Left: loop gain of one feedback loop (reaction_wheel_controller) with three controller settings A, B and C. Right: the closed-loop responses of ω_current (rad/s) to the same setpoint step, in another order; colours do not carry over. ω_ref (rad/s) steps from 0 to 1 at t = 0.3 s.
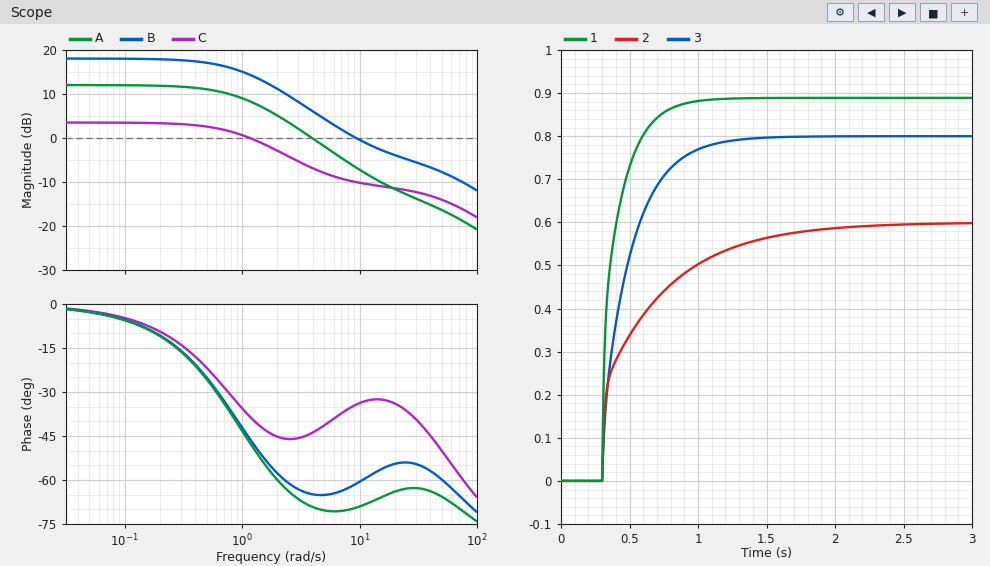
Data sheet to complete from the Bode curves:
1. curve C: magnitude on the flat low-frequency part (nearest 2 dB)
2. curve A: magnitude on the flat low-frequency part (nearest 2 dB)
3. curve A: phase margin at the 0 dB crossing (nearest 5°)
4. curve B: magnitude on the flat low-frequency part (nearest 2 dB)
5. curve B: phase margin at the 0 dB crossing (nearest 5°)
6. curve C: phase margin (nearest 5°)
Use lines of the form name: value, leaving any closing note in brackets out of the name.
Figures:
curve C: magnitude on the flat low-frequency part: 4 dB
curve A: magnitude on the flat low-frequency part: 12 dB
curve A: phase margin at the 0 dB crossing: 110°
curve B: magnitude on the flat low-frequency part: 18 dB
curve B: phase margin at the 0 dB crossing: 120°
curve C: phase margin: 140°
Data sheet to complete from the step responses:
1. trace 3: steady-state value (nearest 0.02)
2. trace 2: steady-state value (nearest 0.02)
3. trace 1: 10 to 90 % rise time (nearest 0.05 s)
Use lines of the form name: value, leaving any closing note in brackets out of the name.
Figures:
trace 3: steady-state value: 0.80
trace 2: steady-state value: 0.60
trace 1: 10 to 90 % rise time: 0.30 s
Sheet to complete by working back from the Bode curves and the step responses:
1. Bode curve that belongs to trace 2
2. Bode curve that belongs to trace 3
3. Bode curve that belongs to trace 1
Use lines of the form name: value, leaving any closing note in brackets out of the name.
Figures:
Bode curve that belongs to trace 2: C
Bode curve that belongs to trace 3: A
Bode curve that belongs to trace 1: B
